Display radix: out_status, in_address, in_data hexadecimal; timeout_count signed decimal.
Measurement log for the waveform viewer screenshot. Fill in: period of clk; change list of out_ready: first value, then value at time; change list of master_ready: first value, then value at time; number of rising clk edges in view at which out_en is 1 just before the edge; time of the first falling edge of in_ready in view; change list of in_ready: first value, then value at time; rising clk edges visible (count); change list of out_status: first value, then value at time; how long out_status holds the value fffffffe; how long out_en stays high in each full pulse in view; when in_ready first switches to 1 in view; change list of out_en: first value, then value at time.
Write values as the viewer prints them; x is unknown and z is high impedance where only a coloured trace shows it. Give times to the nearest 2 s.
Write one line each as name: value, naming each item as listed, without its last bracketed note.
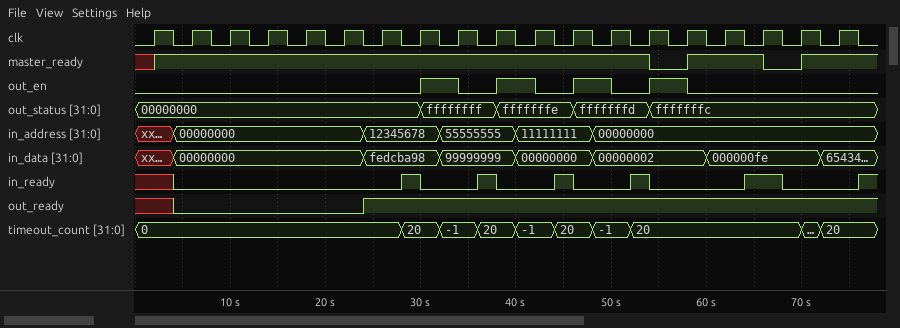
period of clk: 4 s
change list of out_ready: first value, then value at time: x, 0 at 4 s, 1 at 24 s
change list of master_ready: first value, then value at time: x, 1 at 2 s, 0 at 54 s, 1 at 58 s, 0 at 66 s, 1 at 70 s
number of rising clk edges in view at which out_en is 1 just before the edge: 4
time of the first falling edge of in_ready in view: 30 s
change list of in_ready: first value, then value at time: x, 0 at 4 s, 1 at 28 s, 0 at 30 s, 1 at 36 s, 0 at 38 s, 1 at 44 s, 0 at 46 s, 1 at 52 s, 0 at 54 s, 1 at 64 s, 0 at 68 s, 1 at 76 s
rising clk edges visible: 19
change list of out_status: first value, then value at time: 00000000, ffffffff at 30 s, fffffffe at 38 s, fffffffd at 46 s, fffffffc at 54 s
how long out_status holds the value fffffffe: 8 s
how long out_en stays high in each full pulse in view: 4 s, 4 s, 4 s, 4 s
when in_ready first switches to 1 in view: 28 s
change list of out_en: first value, then value at time: 0, 1 at 30 s, 0 at 34 s, 1 at 38 s, 0 at 42 s, 1 at 46 s, 0 at 50 s, 1 at 54 s, 0 at 58 s
